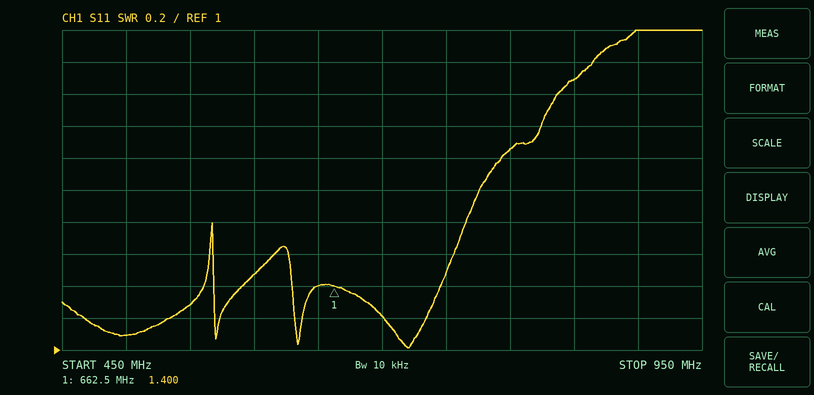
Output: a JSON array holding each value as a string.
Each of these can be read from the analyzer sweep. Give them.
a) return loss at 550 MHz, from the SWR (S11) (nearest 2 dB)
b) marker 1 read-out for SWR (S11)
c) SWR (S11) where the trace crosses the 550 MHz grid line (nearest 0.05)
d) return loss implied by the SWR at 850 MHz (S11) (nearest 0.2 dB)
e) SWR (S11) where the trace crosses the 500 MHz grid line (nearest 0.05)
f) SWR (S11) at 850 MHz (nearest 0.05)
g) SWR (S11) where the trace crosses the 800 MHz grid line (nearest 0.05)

["18 dB", "1.400", "1.30", "6.8 dB", "1.10", "2.70", "2.25"]
